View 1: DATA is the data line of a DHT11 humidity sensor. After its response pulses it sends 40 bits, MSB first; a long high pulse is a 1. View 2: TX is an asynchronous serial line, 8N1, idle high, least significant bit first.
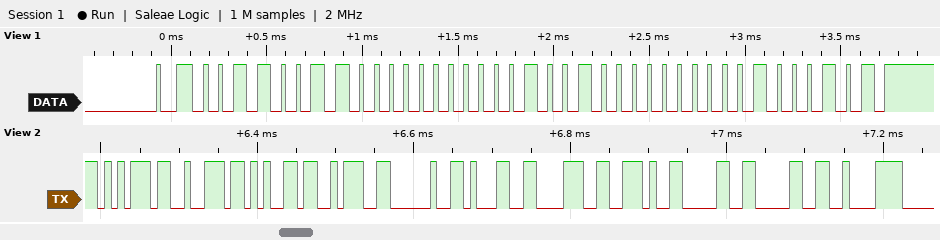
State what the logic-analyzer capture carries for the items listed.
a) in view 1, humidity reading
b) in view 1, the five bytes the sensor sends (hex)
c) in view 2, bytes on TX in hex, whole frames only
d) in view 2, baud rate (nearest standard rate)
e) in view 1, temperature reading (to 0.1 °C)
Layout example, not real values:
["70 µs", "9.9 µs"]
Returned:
["51 %", "33 00 12 00 45", "75 72 65 3A 20 31 38 2E 30 30 C2", "115200 baud", "18.0 °C"]
